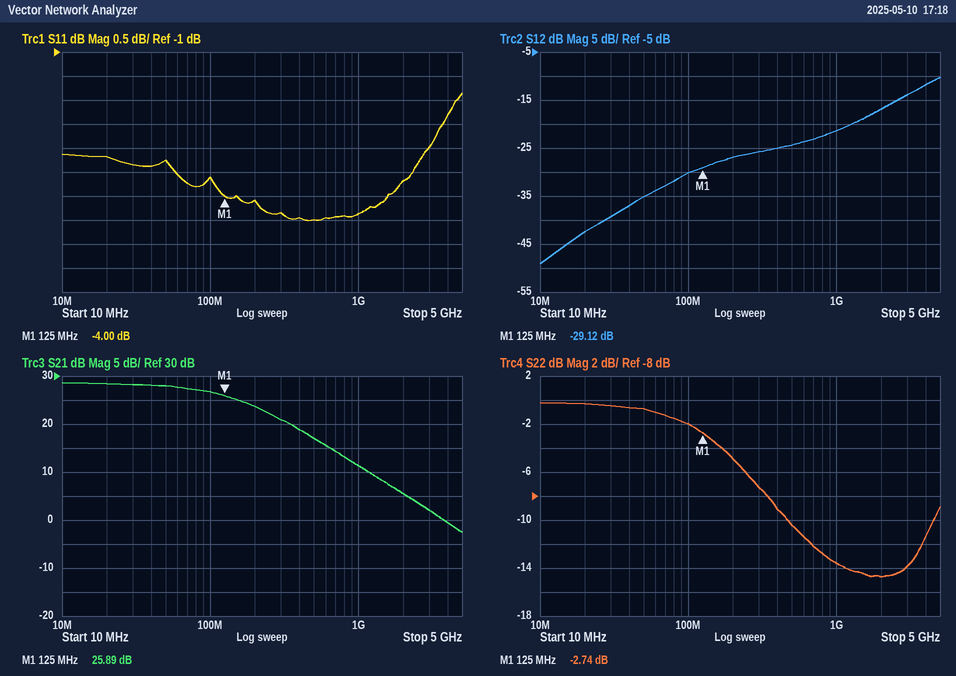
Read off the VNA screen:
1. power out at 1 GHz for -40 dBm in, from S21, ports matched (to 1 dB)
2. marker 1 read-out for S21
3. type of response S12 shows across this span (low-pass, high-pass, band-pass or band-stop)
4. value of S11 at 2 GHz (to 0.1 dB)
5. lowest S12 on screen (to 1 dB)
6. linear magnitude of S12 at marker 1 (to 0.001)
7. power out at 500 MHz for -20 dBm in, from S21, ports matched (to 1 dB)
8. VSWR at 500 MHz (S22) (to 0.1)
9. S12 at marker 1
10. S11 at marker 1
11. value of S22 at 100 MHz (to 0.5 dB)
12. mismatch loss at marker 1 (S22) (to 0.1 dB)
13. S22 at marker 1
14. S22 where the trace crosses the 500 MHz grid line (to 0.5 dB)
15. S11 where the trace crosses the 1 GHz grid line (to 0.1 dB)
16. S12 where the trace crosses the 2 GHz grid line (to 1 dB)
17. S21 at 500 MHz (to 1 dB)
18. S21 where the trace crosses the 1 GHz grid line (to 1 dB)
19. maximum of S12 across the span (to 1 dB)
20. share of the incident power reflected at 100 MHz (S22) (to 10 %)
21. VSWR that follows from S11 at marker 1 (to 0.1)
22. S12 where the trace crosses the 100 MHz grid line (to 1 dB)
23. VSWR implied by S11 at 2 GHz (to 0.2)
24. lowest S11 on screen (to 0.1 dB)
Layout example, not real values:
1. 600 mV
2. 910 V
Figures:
1. -29 dBm
2. 25.89 dB
3. high-pass
4. -3.7 dB
5. -49 dB
6. 0.035
7. -3 dBm
8. 1.9
9. -29.12 dB
10. -4.00 dB
11. -2.0 dB
12. 3.3 dB
13. -2.74 dB
14. -10.5 dB
15. -4.4 dB
16. -17 dB
17. 17 dB
18. 11 dB
19. -10 dB
20. 60 %
21. 4.4
22. -30 dB
23. 4.8
24. -4.5 dB
